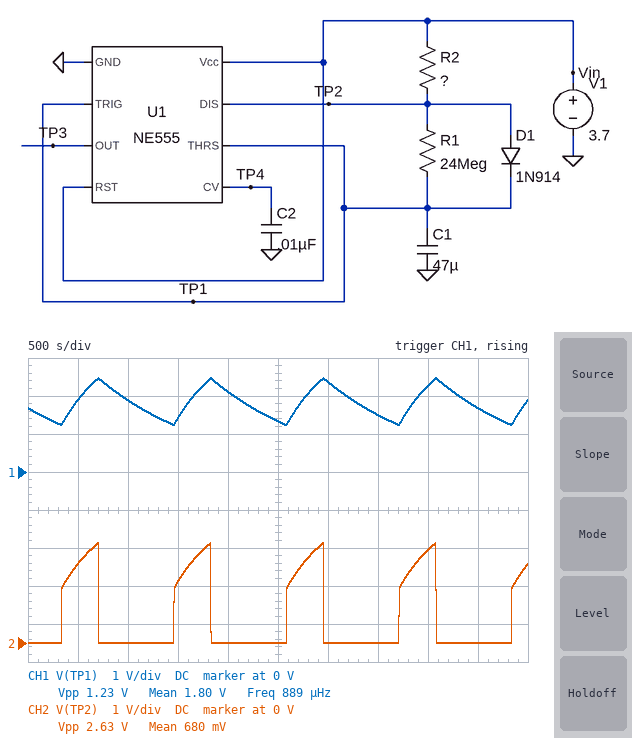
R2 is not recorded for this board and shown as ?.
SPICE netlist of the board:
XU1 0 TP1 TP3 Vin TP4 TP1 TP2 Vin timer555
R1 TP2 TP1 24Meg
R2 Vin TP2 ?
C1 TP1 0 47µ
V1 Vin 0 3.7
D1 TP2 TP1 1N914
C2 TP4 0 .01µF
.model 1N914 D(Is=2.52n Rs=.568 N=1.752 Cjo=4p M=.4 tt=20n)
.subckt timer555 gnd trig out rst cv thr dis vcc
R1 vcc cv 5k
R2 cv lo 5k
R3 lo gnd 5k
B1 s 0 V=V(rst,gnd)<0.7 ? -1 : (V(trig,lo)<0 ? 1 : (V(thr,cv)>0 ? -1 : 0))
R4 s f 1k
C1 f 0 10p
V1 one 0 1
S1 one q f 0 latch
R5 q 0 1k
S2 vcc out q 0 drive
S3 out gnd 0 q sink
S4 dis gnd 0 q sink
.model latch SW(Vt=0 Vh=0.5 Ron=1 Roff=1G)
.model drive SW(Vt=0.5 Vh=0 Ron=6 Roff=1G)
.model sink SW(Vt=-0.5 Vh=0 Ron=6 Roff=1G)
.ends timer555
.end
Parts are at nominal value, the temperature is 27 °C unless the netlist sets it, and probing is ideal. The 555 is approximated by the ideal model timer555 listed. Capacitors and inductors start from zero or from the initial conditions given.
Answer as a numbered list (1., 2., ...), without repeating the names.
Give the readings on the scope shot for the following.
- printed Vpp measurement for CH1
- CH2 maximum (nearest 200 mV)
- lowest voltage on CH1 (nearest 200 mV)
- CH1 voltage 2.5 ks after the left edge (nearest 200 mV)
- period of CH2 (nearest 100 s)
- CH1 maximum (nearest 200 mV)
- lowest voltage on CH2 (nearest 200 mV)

1. 1.23 V
2. 2.6 V
3. 1.2 V
4. 1.4 V
5. 1.1 ks
6. 2.4 V
7. 0 V
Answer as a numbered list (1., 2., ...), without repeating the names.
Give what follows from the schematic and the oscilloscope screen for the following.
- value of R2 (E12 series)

1. 10 MΩ
